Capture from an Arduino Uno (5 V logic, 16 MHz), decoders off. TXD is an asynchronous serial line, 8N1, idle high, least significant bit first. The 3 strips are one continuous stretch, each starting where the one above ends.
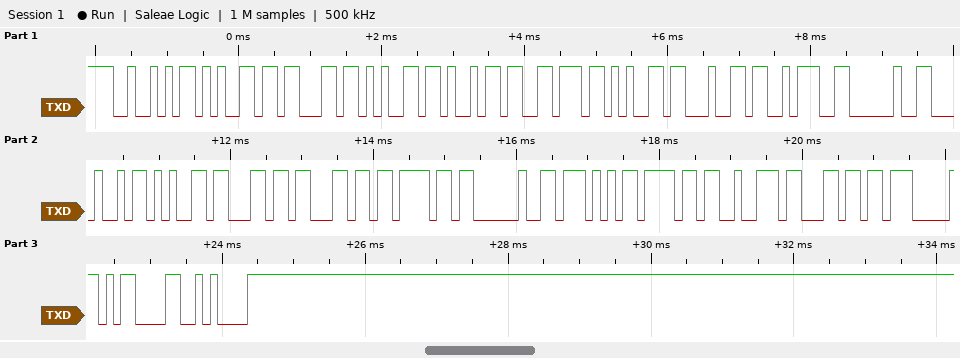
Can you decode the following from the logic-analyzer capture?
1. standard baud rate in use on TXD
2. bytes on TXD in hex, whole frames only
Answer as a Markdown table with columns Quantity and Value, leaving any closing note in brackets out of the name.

| Quantity | Value |
|---|---|
| standard baud rate in use on TXD | 9600 baud |
| bytes on TXD in hex, whole frames only | 0x52 0x65 0x63 0x65 0x69 0x76 0x65 0x64 0x3A 0x20 0x48 0x65 0x6C 0x6C 0x6F 0x20 0x57 0x6F 0x72 0x6C 0x07 0x0D 0x0A |
